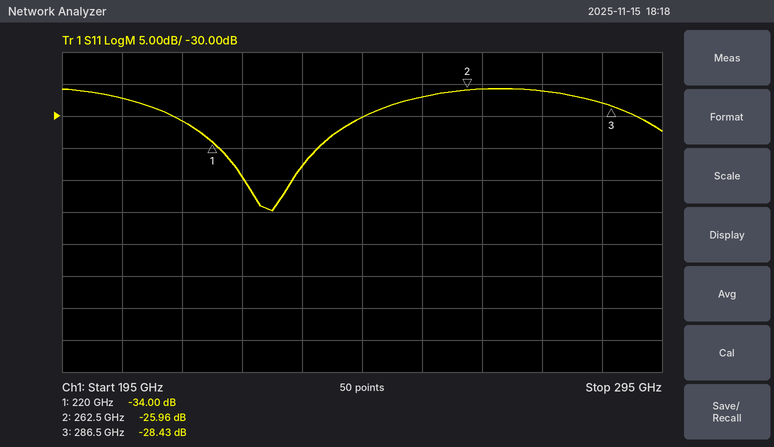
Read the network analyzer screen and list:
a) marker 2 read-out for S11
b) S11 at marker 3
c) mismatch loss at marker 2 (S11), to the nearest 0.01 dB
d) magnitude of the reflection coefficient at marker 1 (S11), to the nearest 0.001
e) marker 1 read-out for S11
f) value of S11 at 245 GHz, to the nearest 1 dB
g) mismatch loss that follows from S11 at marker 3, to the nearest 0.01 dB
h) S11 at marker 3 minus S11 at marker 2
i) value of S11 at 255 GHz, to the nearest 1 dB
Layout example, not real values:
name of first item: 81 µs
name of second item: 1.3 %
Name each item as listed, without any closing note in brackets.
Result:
marker 2 read-out for S11: -25.96 dB
S11 at marker 3: -28.43 dB
mismatch loss at marker 2 (S11), to the nearest 0.01 dB: 0.01 dB
magnitude of the reflection coefficient at marker 1 (S11), to the nearest 0.001: 0.020
marker 1 read-out for S11: -34.00 dB
value of S11 at 245 GHz, to the nearest 1 dB: -30 dB
mismatch loss that follows from S11 at marker 3, to the nearest 0.01 dB: 0.01 dB
S11 at marker 3 minus S11 at marker 2: -2.47 dB
value of S11 at 255 GHz, to the nearest 1 dB: -27 dB
